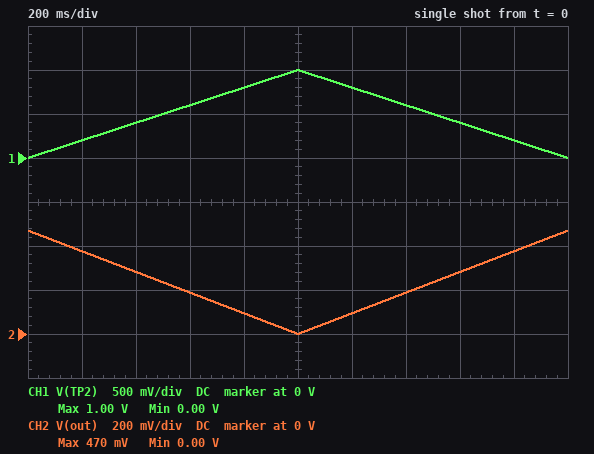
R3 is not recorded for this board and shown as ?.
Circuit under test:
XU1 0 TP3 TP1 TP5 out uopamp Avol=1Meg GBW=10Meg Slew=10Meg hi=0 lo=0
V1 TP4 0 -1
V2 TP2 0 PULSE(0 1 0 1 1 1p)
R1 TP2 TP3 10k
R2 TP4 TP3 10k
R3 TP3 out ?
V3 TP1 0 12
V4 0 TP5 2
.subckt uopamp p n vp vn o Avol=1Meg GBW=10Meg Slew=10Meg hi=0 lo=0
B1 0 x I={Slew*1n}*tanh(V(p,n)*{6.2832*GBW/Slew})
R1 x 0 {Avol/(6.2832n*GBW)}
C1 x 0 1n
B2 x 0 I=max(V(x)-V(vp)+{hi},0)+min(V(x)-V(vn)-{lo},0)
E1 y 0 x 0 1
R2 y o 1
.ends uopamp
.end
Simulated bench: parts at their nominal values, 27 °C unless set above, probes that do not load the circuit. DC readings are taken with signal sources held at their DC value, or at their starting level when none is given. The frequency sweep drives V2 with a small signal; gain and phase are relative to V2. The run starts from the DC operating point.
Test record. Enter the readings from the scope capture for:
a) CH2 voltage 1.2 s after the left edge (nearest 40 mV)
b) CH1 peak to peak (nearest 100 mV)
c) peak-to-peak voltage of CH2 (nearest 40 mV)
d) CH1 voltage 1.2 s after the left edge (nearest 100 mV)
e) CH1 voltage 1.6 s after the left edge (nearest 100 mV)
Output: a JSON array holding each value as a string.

["80 mV", "1.0 V", "480 mV", "800 mV", "400 mV"]
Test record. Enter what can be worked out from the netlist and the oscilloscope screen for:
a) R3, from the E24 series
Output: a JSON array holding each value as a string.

["4.7 kΩ"]
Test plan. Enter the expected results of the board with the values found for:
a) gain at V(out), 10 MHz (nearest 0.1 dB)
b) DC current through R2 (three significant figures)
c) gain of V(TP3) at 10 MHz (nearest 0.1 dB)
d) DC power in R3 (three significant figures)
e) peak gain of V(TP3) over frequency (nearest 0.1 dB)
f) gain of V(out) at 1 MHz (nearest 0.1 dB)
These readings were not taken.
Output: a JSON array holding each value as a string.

["-13.3 dB", "100 µA", "-13.3 dB", "47.0 µW", "-12.3 dB", "-6.7 dB"]
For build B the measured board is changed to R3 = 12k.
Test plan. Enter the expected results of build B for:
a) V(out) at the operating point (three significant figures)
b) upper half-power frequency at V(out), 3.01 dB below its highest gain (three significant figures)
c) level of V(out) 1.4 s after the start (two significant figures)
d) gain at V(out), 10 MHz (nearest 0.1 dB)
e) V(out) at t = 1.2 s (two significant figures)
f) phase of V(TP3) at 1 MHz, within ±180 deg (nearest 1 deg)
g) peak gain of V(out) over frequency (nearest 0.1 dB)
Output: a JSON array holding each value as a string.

["1.20 V", "2.94 MHz", "480 mV", "-9.4 dB", "240 mV", "71 deg", "1.6 dB"]
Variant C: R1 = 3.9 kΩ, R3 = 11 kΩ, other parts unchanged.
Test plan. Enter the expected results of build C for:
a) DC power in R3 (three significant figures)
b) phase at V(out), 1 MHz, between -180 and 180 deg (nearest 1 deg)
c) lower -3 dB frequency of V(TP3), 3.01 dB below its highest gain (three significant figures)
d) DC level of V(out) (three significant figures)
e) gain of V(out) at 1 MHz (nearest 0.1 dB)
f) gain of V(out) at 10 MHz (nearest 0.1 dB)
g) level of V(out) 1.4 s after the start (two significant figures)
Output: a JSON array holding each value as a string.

["110 µW", "154 deg", "2.03 MHz", "1.10 V", "8.1 dB", "-5.0 dB", "-590 mV"]
